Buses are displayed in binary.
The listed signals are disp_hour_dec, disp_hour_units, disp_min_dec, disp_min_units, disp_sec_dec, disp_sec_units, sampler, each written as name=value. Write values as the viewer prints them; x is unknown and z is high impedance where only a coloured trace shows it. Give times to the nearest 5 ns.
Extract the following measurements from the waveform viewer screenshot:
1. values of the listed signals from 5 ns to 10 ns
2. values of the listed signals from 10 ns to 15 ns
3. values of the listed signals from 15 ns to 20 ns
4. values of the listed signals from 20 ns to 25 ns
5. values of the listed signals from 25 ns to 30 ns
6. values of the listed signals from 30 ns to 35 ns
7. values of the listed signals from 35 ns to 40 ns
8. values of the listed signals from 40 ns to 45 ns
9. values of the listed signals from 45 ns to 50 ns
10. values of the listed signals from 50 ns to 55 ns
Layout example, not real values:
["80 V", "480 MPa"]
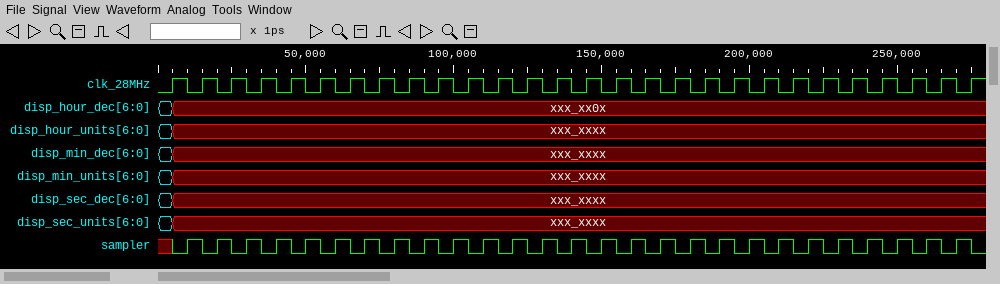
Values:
["disp_hour_dec=xxx_xx0x, disp_hour_units=xxx_xxxx, disp_min_dec=xxx_xxxx, disp_min_units=xxx_xxxx, disp_sec_dec=xxx_xxxx, disp_sec_units=xxx_xxxx, sampler=0", "disp_hour_dec=xxx_xx0x, disp_hour_units=xxx_xxxx, disp_min_dec=xxx_xxxx, disp_min_units=xxx_xxxx, disp_sec_dec=xxx_xxxx, disp_sec_units=xxx_xxxx, sampler=1", "disp_hour_dec=xxx_xx0x, disp_hour_units=xxx_xxxx, disp_min_dec=xxx_xxxx, disp_min_units=xxx_xxxx, disp_sec_dec=xxx_xxxx, disp_sec_units=xxx_xxxx, sampler=0", "disp_hour_dec=xxx_xx0x, disp_hour_units=xxx_xxxx, disp_min_dec=xxx_xxxx, disp_min_units=xxx_xxxx, disp_sec_dec=xxx_xxxx, disp_sec_units=xxx_xxxx, sampler=1", "disp_hour_dec=xxx_xx0x, disp_hour_units=xxx_xxxx, disp_min_dec=xxx_xxxx, disp_min_units=xxx_xxxx, disp_sec_dec=xxx_xxxx, disp_sec_units=xxx_xxxx, sampler=0", "disp_hour_dec=xxx_xx0x, disp_hour_units=xxx_xxxx, disp_min_dec=xxx_xxxx, disp_min_units=xxx_xxxx, disp_sec_dec=xxx_xxxx, disp_sec_units=xxx_xxxx, sampler=1", "disp_hour_dec=xxx_xx0x, disp_hour_units=xxx_xxxx, disp_min_dec=xxx_xxxx, disp_min_units=xxx_xxxx, disp_sec_dec=xxx_xxxx, disp_sec_units=xxx_xxxx, sampler=0", "disp_hour_dec=xxx_xx0x, disp_hour_units=xxx_xxxx, disp_min_dec=xxx_xxxx, disp_min_units=xxx_xxxx, disp_sec_dec=xxx_xxxx, disp_sec_units=xxx_xxxx, sampler=1", "disp_hour_dec=xxx_xx0x, disp_hour_units=xxx_xxxx, disp_min_dec=xxx_xxxx, disp_min_units=xxx_xxxx, disp_sec_dec=xxx_xxxx, disp_sec_units=xxx_xxxx, sampler=0", "disp_hour_dec=xxx_xx0x, disp_hour_units=xxx_xxxx, disp_min_dec=xxx_xxxx, disp_min_units=xxx_xxxx, disp_sec_dec=xxx_xxxx, disp_sec_units=xxx_xxxx, sampler=1"]
